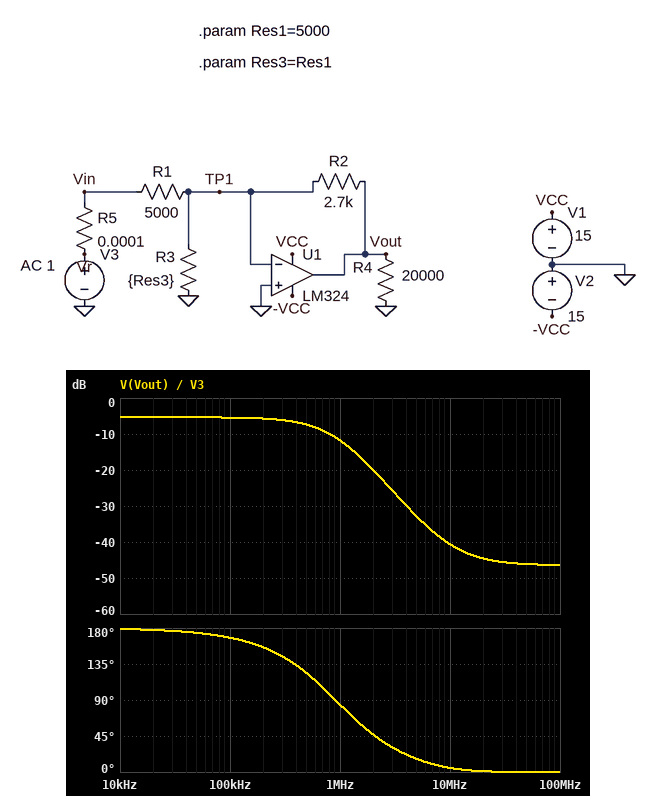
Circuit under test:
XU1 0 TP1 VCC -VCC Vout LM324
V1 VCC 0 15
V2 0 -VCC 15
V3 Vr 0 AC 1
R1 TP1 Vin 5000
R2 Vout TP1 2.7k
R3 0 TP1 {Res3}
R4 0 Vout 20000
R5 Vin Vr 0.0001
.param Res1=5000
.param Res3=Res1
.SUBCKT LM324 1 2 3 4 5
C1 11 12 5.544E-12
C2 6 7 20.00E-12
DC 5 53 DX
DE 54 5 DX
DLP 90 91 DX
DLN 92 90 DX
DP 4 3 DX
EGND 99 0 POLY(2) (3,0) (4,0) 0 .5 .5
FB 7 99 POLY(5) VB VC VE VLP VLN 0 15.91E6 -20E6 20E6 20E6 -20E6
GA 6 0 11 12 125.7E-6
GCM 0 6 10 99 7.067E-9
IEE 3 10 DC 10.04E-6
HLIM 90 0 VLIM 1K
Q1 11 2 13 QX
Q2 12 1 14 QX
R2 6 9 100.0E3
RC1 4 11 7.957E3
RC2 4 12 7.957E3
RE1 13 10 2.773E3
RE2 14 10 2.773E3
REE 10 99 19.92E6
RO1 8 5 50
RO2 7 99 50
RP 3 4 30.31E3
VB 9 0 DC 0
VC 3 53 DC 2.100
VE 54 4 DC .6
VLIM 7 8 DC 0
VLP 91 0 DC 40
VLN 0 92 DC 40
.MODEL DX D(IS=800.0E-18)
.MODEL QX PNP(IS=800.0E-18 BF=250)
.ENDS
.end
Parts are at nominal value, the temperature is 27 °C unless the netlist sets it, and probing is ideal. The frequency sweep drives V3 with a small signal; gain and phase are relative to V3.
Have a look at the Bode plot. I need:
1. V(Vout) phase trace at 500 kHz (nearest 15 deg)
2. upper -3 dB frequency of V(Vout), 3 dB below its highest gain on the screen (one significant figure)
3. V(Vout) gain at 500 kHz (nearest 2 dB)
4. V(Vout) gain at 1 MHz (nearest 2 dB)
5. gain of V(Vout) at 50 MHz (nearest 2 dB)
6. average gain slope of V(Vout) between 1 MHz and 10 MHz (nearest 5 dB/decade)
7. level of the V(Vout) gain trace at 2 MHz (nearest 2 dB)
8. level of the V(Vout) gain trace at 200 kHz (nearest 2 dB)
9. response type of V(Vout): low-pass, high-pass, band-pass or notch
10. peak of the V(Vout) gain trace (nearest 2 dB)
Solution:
120 deg
600 kHz
-8 dB
-12 dB
-46 dB
-30 dB/decade
-20 dB
-6 dB
low-pass
-6 dB
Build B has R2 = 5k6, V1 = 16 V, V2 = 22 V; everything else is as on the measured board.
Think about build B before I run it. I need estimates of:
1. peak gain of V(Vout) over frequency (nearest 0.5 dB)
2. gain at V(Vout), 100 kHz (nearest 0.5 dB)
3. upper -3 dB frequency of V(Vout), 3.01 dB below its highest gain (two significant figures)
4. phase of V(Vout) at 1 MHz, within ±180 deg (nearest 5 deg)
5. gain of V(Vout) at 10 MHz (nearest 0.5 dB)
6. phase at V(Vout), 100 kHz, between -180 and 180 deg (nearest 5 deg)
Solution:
1.0 dB
0.5 dB
360 kHz
75 deg
-41.0 dB
160 deg
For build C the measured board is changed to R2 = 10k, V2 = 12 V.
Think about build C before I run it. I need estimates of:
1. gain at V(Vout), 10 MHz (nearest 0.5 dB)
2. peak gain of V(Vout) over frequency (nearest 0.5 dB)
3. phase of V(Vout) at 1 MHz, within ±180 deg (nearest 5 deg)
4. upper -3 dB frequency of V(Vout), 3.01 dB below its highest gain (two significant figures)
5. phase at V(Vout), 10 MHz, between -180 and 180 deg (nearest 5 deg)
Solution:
-41.0 dB
6.0 dB
70 deg
220 kHz
10 deg
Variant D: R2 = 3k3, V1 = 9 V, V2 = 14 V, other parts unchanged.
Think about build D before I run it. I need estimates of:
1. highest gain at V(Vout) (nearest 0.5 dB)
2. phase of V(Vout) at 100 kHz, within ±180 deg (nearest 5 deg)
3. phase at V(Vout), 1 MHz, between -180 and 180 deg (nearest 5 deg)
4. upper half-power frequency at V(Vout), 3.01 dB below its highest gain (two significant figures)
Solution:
-3.5 dB
165 deg
80 deg
540 kHz
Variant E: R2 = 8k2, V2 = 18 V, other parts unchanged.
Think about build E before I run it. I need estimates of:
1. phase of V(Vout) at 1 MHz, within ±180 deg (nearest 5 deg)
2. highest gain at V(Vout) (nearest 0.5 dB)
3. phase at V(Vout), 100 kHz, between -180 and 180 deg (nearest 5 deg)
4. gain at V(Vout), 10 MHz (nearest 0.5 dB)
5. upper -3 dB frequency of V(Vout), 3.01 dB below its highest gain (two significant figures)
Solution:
70 deg
4.5 dB
155 deg
-41.0 dB
260 kHz
